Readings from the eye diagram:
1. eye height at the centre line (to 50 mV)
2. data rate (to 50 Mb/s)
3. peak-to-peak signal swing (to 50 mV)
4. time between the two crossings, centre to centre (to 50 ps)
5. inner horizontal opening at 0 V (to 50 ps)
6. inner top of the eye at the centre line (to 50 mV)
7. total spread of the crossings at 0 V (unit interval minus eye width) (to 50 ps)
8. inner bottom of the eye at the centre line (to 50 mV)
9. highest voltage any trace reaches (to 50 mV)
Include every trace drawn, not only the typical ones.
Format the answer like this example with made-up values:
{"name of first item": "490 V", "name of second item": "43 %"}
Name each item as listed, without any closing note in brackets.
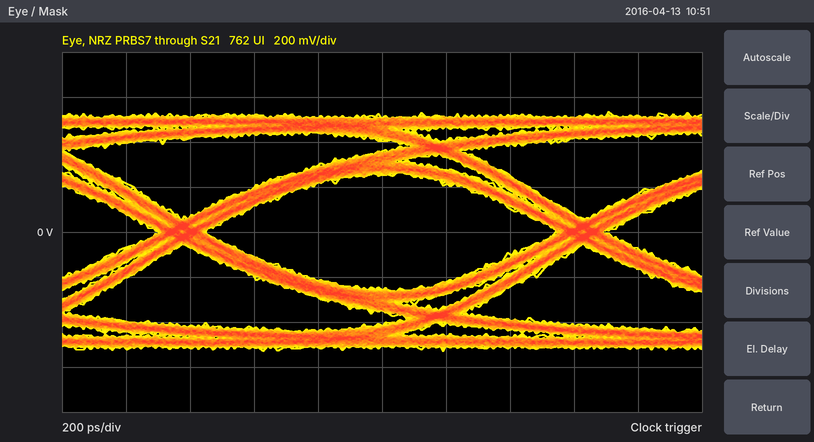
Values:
{"eye height at the centre line": "500 mV", "data rate": "800 Mb/s", "peak-to-peak signal swing": "1.05 V", "time between the two crossings, centre to centre": "1.25 ns", "inner horizontal opening at 0 V": "1.10 ns", "inner top of the eye at the centre line": "250 mV", "total spread of the crossings at 0 V (unit interval minus eye width)": "150 ps", "inner bottom of the eye at the centre line": "-250 mV", "highest voltage any trace reaches": "550 mV"}
